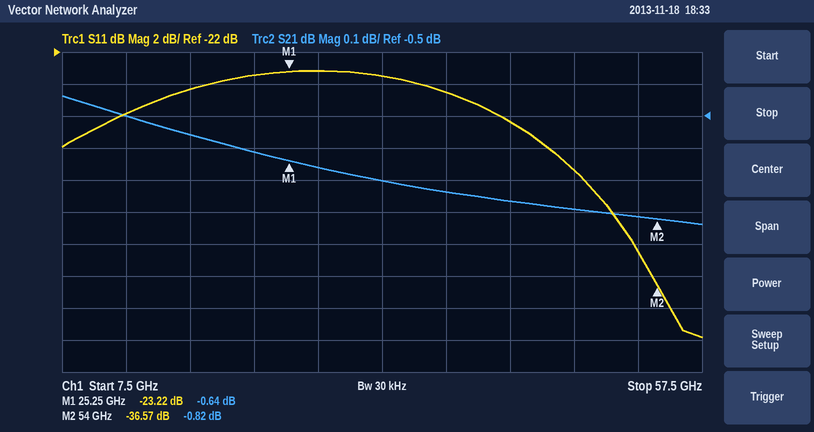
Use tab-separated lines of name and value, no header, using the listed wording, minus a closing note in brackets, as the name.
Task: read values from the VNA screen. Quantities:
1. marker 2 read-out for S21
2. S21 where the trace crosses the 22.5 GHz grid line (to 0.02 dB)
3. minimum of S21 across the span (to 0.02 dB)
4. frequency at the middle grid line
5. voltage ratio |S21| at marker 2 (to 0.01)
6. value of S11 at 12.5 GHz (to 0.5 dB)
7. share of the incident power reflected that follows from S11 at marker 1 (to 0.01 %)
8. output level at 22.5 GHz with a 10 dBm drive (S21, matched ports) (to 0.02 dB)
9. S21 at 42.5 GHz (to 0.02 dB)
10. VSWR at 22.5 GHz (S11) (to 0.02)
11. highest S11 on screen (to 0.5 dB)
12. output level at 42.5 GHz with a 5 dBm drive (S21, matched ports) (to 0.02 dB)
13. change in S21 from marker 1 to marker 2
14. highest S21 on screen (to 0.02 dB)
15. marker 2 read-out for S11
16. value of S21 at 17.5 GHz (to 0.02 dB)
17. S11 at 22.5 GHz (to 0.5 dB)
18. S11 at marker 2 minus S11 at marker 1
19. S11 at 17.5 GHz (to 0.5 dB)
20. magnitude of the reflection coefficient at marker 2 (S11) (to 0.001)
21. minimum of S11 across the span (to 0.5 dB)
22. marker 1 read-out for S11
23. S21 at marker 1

marker 2 read-out for S21	-0.82 dB
S21 where the trace crosses the 22.5 GHz grid line	-0.62 dB
minimum of S21 across the span	-0.84 dB
frequency at the middle grid line	32.5 GHz
voltage ratio |S21| at marker 2	0.91
value of S11 at 12.5 GHz	-26.0 dB
share of the incident power reflected that follows from S11 at marker 1	0.48 %
output level at 22.5 GHz with a 10 dBm drive (S21, matched ports)	9.38 dBm
S21 at 42.5 GHz	-0.76 dB
VSWR at 22.5 GHz (S11)	1.14
highest S11 on screen	-23.0 dB
output level at 42.5 GHz with a 5 dBm drive (S21, matched ports)	4.24 dBm
change in S21 from marker 1 to marker 2	-0.18 dB
highest S21 on screen	-0.44 dB
marker 2 read-out for S11	-36.57 dB
value of S21 at 17.5 GHz	-0.56 dB
S11 at 22.5 GHz	-23.5 dB
S11 at marker 2 minus S11 at marker 1	-13.35 dB
S11 at 17.5 GHz	-24.5 dB
magnitude of the reflection coefficient at marker 2 (S11)	0.015
minimum of S11 across the span	-40.0 dB
marker 1 read-out for S11	-23.22 dB
S21 at marker 1	-0.64 dB
